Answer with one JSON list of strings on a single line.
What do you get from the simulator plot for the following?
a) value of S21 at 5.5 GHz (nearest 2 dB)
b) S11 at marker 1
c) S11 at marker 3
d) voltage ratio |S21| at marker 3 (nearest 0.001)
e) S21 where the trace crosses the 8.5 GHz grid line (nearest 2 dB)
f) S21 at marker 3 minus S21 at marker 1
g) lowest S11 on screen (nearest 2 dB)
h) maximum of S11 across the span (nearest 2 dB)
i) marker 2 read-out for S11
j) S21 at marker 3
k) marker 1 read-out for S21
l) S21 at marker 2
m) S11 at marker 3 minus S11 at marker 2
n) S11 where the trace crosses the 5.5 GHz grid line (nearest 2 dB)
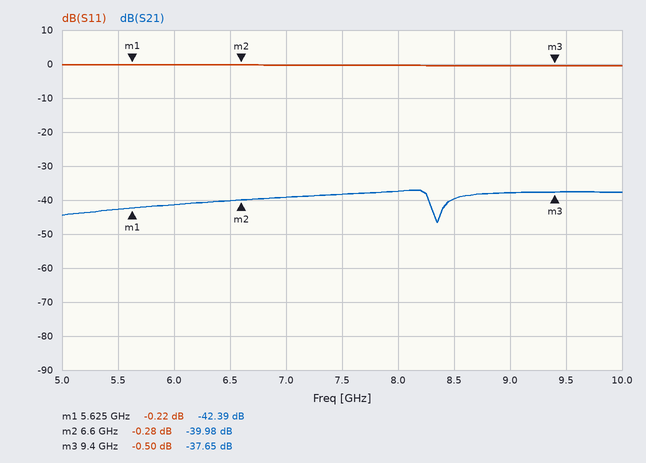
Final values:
["-42 dB", "-0.22 dB", "-0.50 dB", "0.013", "-40 dB", "4.74 dB", "0 dB", "0 dB", "-0.28 dB", "-37.65 dB", "-42.39 dB", "-39.98 dB", "-0.22 dB", "0 dB"]
